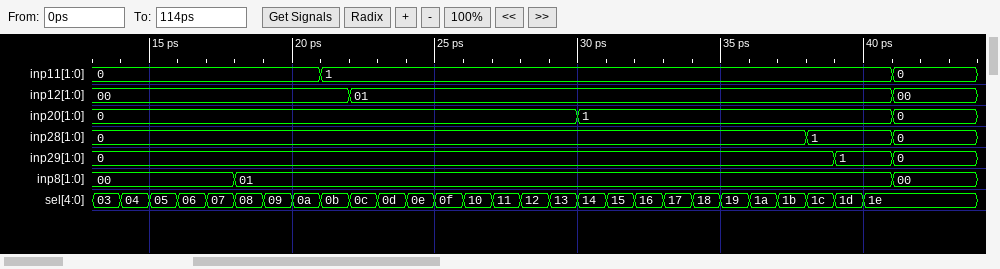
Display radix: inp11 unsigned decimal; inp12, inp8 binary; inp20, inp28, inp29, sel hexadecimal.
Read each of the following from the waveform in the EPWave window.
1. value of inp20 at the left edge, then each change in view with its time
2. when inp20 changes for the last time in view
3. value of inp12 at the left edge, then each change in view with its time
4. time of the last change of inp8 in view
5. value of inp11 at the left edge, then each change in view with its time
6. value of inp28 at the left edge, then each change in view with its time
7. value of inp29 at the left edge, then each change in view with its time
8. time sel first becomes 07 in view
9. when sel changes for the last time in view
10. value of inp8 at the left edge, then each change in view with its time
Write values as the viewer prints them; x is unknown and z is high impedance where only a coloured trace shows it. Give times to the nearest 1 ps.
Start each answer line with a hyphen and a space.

- 0, 1 at 30 ps, 0 at 41 ps
- 41 ps
- 00, 01 at 22 ps, 00 at 41 ps
- 41 ps
- 0, 1 at 21 ps, 0 at 41 ps
- 0, 1 at 38 ps, 0 at 41 ps
- 0, 1 at 39 ps, 0 at 41 ps
- 17 ps
- 40 ps
- 00, 01 at 18 ps, 00 at 41 ps
